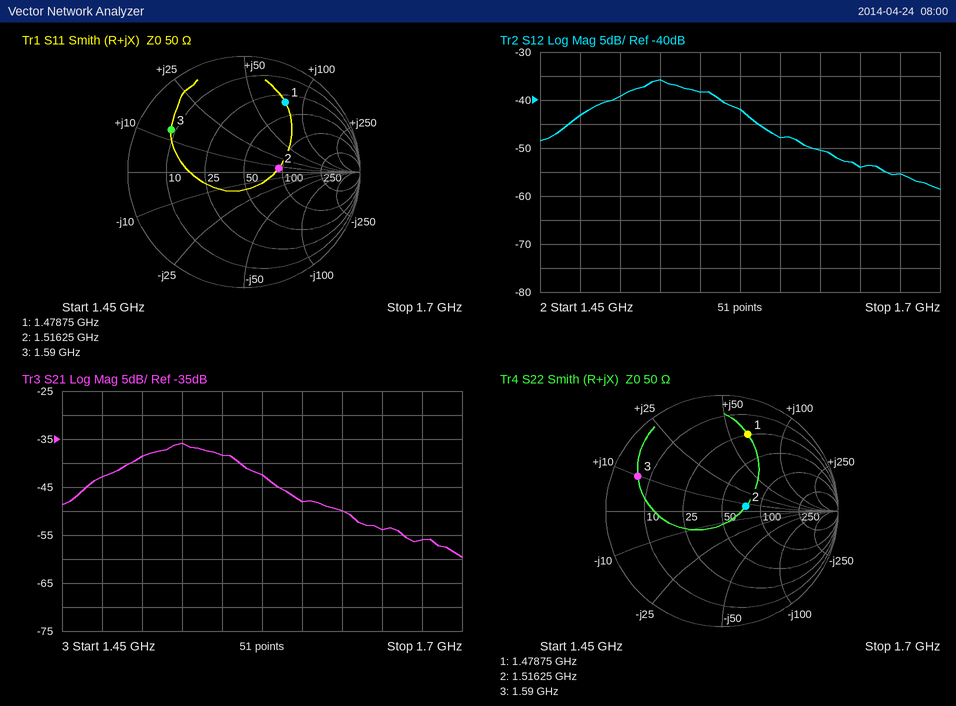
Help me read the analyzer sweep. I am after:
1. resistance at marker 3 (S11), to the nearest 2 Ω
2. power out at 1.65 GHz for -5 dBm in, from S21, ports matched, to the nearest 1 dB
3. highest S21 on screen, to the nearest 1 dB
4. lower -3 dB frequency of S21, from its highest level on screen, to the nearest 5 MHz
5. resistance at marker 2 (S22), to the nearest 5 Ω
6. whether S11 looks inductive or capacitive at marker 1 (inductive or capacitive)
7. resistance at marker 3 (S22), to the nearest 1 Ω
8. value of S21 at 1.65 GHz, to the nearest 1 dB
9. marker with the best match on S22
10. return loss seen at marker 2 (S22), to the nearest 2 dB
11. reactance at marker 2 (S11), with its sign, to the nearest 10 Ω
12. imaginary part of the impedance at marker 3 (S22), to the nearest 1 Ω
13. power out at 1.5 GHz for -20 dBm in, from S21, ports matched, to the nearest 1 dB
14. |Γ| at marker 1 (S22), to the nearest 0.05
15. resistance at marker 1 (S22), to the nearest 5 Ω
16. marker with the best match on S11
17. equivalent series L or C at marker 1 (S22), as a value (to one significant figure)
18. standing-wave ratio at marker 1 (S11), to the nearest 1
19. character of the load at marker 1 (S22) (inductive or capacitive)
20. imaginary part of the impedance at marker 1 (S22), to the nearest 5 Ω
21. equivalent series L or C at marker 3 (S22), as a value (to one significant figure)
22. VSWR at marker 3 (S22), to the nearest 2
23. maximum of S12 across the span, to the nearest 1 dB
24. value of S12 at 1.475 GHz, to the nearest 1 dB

8 Ω
-59 dBm
-36 dB
1.500 GHz
75 Ω
inductive
6 Ω
-54 dB
marker 2
14 dB
+10 Ω
+10 Ω
-59 dBm
0.70
25 Ω
marker 2
7 nH
6
inductive
+65 Ω
1.0 nH
8
-36 dB
-43 dB
